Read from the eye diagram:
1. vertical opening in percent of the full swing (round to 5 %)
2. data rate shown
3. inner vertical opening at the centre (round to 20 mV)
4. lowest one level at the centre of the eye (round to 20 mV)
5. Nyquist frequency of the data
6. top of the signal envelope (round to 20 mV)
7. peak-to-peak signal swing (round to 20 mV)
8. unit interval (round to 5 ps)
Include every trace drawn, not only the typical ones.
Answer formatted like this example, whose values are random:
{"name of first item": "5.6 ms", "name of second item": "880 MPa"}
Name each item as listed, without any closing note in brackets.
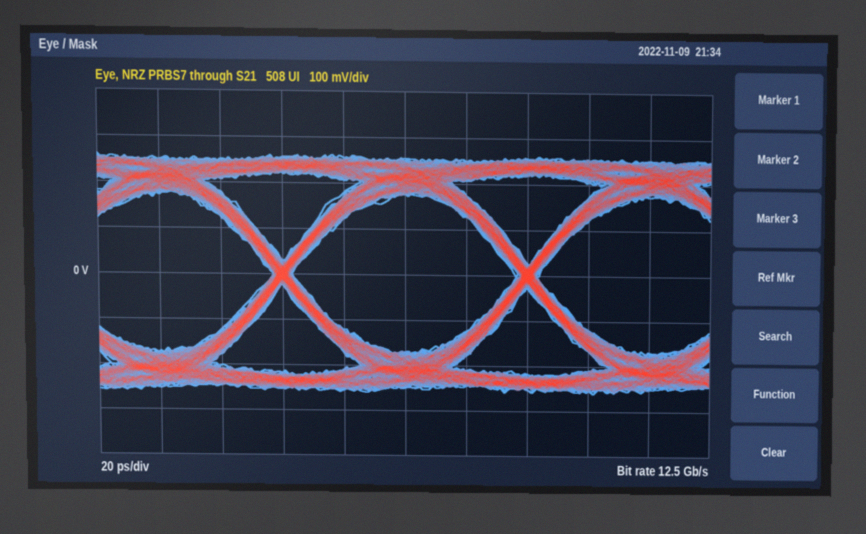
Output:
{"vertical opening in percent of the full swing": "65 %", "data rate shown": "12.5 Gb/s", "inner vertical opening at the centre": "340 mV", "lowest one level at the centre of the eye": "180 mV", "Nyquist frequency of the data": "6.25 GHz", "top of the signal envelope": "260 mV", "peak-to-peak signal swing": "520 mV", "unit interval": "80 ps"}
